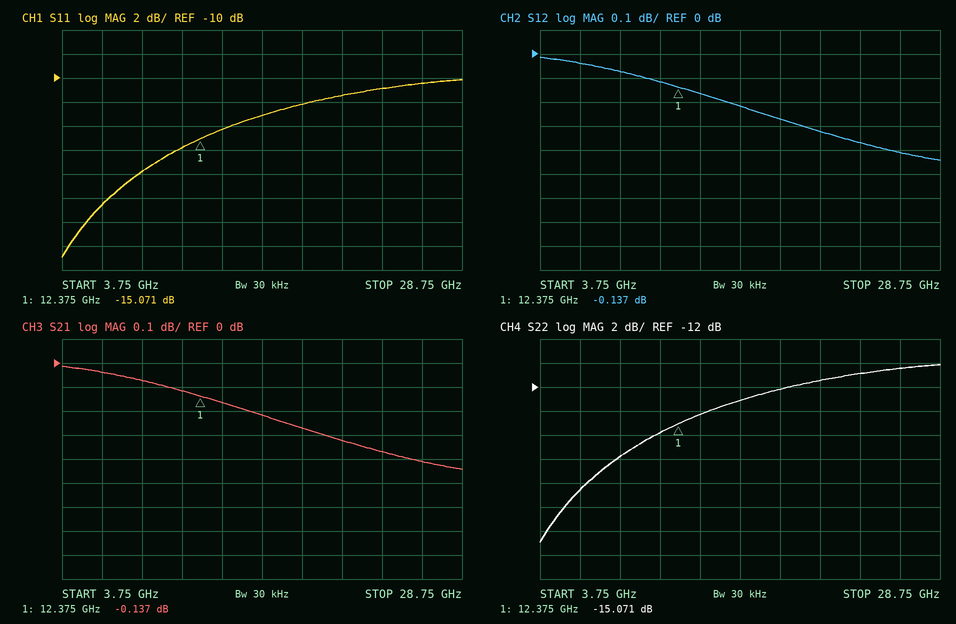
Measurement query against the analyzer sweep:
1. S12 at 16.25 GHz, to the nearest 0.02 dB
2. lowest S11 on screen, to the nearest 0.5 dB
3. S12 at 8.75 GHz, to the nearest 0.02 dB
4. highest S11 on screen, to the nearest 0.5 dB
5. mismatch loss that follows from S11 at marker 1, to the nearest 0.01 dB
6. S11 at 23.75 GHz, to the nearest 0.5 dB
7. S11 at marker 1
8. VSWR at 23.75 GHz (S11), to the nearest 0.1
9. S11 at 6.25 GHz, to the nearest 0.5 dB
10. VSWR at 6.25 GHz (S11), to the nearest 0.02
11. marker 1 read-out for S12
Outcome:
-0.22 dB
-25.0 dB
-0.08 dB
-10.0 dB
0.14 dB
-11.0 dB
-15.071 dB
1.8
-20.5 dB
1.20
-0.137 dB
